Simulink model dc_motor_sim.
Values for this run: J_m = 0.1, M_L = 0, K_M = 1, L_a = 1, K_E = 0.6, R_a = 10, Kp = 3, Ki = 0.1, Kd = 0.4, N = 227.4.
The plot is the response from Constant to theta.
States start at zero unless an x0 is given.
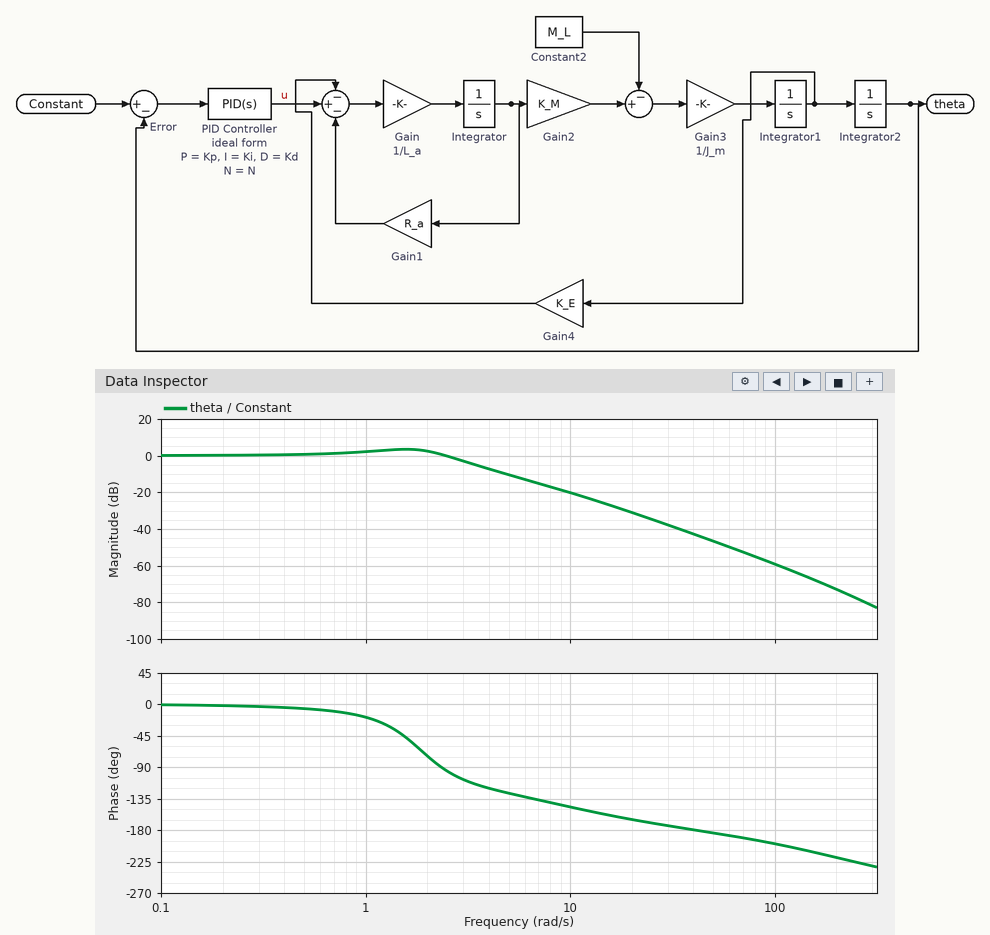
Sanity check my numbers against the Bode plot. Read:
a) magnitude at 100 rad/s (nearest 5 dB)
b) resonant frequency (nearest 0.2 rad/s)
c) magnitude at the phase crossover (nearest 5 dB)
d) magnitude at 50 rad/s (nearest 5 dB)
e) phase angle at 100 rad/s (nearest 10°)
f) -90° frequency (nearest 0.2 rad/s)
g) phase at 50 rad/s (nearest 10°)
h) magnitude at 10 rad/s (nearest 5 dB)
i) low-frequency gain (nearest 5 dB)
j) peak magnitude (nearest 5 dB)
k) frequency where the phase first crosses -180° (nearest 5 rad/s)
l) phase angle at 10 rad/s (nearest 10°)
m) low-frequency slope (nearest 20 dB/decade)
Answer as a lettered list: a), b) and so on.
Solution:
a) -60 dB
b) 1.6 rad/s
c) -45 dB
d) -45 dB
e) -200°
f) 2.4 rad/s
g) -180°
h) -20 dB
i) 0 dB
j) 5 dB
k) 40 rad/s
l) -150°
m) 0 dB/decade
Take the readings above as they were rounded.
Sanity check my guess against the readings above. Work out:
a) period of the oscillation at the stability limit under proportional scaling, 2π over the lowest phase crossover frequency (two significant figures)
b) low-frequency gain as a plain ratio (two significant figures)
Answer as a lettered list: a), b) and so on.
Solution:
a) 0.16 s
b) 1.0
